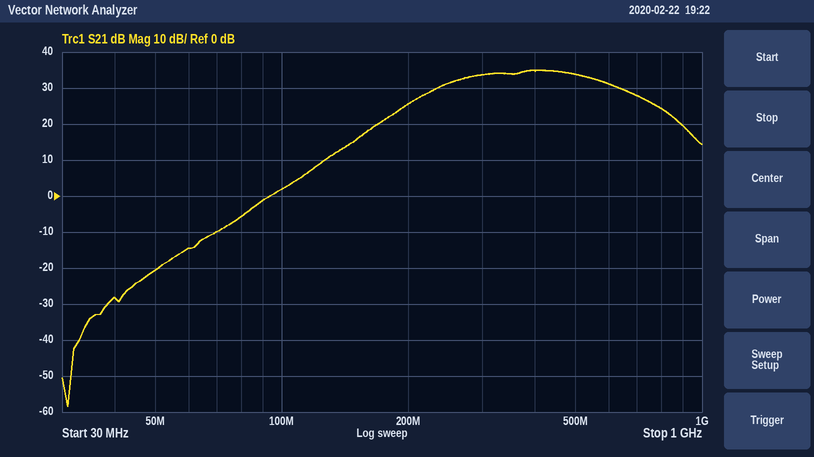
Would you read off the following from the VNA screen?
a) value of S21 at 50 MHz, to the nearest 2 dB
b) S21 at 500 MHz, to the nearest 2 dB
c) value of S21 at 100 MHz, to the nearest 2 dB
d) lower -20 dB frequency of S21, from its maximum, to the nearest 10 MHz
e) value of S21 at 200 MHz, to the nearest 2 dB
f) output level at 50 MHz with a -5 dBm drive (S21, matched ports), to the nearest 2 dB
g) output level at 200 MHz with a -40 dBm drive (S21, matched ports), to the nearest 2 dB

-20 dB
34 dB
2 dB
150 MHz
26 dB
-26 dBm
-14 dBm
